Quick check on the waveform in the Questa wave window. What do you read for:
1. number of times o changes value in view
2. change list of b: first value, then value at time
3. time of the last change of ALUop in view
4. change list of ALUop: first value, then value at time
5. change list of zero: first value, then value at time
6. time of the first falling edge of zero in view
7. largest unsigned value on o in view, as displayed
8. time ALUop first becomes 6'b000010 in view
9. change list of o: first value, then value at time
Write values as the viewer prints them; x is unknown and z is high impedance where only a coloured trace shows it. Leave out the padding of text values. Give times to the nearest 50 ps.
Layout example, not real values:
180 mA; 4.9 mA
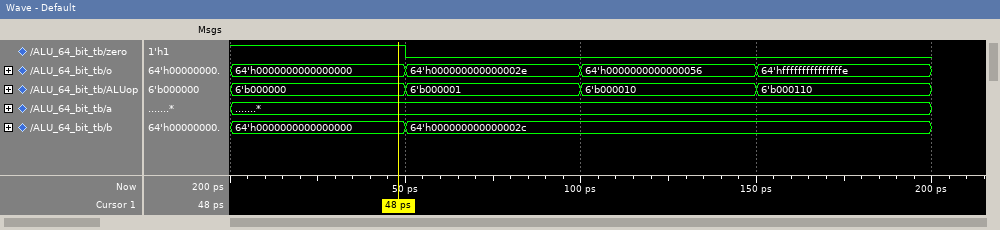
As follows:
3; 64'h0000000000000000, 64'h000000000000002c at 50 ps; 150 ps; 6'b000000, 6'b000001 at 50 ps, 6'b000010 at 100 ps, 6'b000110 at 150 ps; 1, 0 at 50 ps; 50 ps; 64'hfffffffffffffffe; 100 ps; 64'h0000000000000000, 64'h000000000000002e at 50 ps, 64'h0000000000000056 at 100 ps, 64'hfffffffffffffffe at 150 ps
